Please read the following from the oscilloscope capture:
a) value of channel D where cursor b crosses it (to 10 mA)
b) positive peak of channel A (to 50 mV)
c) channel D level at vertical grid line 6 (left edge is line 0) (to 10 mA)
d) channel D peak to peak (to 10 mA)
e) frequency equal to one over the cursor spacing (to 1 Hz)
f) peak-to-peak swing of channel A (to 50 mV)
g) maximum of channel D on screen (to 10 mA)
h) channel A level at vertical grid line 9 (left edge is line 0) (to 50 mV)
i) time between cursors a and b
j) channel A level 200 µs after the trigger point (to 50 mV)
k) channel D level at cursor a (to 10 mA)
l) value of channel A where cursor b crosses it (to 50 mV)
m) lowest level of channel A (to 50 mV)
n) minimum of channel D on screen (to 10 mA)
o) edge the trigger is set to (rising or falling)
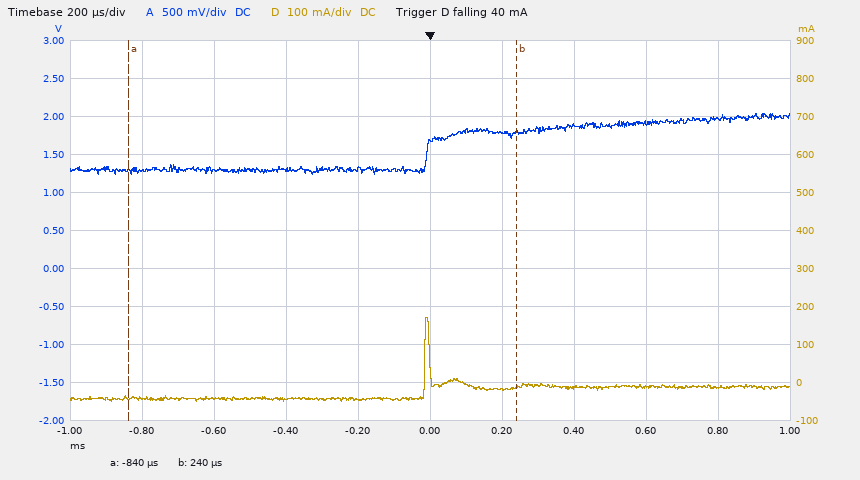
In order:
-10 mA
2.05 V
-20 mA
220 mA
926 Hz
800 mV
170 mA
1.95 V
1.08 ms
1.80 V
-40 mA
1.80 V
1.25 V
-50 mA
falling
